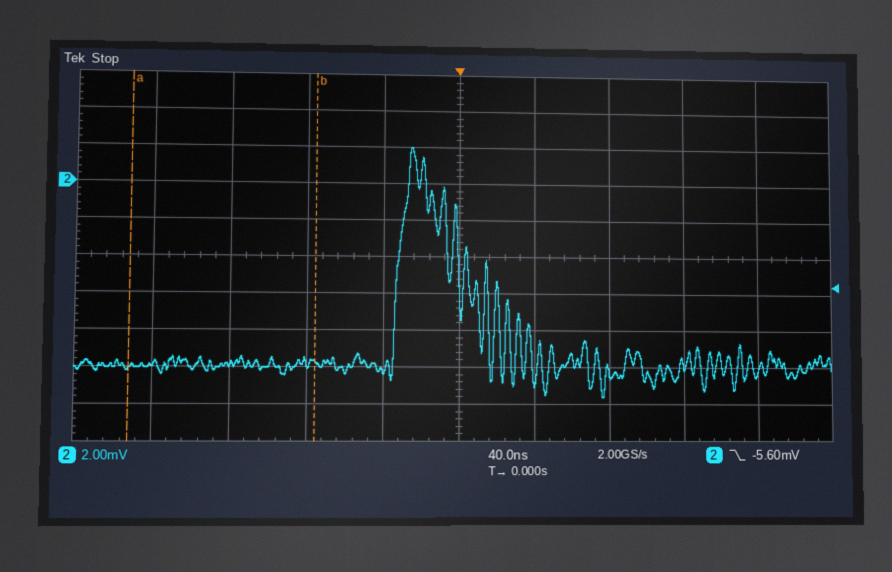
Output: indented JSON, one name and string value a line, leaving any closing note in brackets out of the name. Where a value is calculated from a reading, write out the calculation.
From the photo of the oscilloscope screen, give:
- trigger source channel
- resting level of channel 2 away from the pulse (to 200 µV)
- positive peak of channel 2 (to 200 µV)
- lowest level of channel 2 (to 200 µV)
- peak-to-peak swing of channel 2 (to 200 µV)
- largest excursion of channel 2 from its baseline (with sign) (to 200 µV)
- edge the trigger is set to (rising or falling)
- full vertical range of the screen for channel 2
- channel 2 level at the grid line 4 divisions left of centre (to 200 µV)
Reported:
{
  "trigger source channel": "channel 2",
  "resting level of channel 2 away from the pulse": "-9.8 mV",
  "positive peak of channel 2": "2.0 mV",
  "lowest level of channel 2": "-11.6 mV",
  "peak-to-peak swing of channel 2": "2.0 mV − (-11.6 mV) = 13.6 mV",
  "largest excursion of channel 2 from its baseline (with sign)": "2.0 mV − (-9.8 mV) = +11.8 mV",
  "edge the trigger is set to": "falling",
  "full vertical range of the screen for channel 2": "20 mV",
  "channel 2 level at the grid line 4 divisions left of centre": "-9.8 mV"
}
